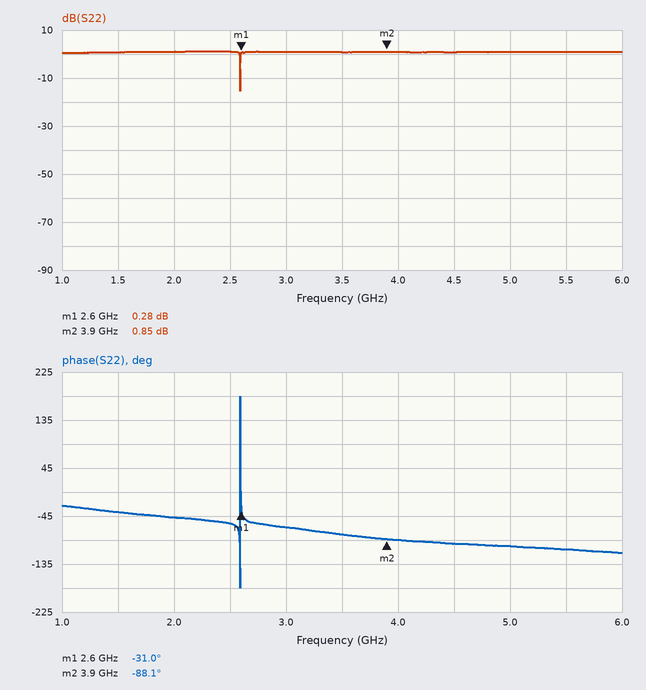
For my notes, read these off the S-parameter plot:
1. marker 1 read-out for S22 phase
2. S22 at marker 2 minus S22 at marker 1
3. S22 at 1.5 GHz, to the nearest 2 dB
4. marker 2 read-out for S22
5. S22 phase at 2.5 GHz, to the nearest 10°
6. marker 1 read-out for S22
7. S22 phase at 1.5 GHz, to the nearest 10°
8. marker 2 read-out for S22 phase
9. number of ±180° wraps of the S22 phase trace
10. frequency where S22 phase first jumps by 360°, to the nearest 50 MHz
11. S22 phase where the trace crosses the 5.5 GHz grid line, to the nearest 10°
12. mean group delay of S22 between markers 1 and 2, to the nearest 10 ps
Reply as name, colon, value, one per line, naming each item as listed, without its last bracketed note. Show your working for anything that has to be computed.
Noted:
marker 1 read-out for S22 phase: -31.0°
S22 at marker 2 minus S22 at marker 1: 0.85 − (0.28) = 0.57 dB
S22 at 1.5 GHz, to the nearest 2 dB: 0 dB
marker 2 read-out for S22: 0.85 dB
S22 phase at 2.5 GHz, to the nearest 10°: -60°
marker 1 read-out for S22: 0.28 dB
S22 phase at 1.5 GHz, to the nearest 10°: -40°
marker 2 read-out for S22 phase: -88.1°
number of ±180° wraps of the S22 phase trace: 1
frequency where S22 phase first jumps by 360°, to the nearest 50 MHz: 2.60 GHz
S22 phase where the trace crosses the 5.5 GHz grid line, to the nearest 10°: -110°
mean group delay of S22 between markers 1 and 2, to the nearest 10 ps: −(-88.1° − (-31°))/(360° × 1.3 GHz) ≈ 122 ps, so 120 ps to the nearest 10 ps
